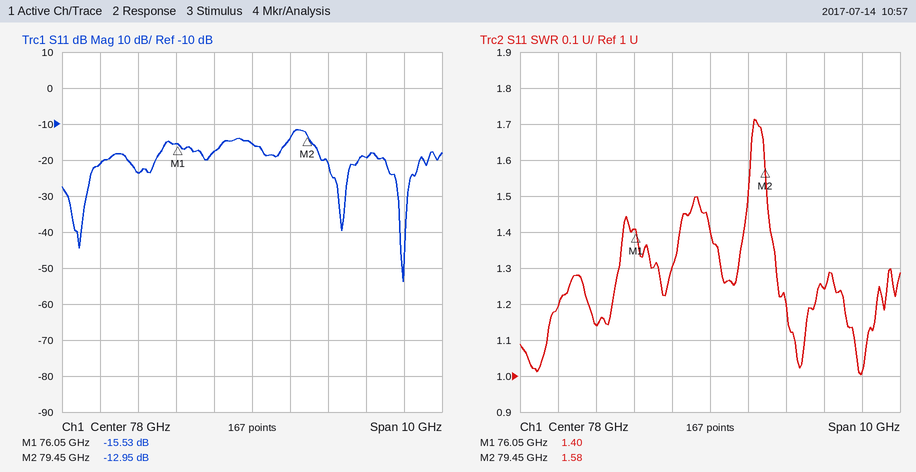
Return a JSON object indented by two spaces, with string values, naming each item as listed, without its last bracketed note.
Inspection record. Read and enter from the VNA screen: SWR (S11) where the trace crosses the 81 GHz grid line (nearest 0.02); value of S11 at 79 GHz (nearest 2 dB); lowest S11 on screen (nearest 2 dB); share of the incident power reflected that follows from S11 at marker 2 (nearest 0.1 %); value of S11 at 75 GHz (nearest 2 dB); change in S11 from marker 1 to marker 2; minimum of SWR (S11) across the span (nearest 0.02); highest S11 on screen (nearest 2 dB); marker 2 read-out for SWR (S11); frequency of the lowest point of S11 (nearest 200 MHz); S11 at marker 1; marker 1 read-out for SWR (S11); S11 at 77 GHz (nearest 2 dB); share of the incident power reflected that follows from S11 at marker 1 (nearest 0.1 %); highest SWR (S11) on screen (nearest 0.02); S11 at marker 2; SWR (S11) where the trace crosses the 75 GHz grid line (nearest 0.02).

{
  "SWR (S11) where the trace crosses the 81 GHz grid line": "1.24",
  "value of S11 at 79 GHz": "-14 dB",
  "lowest S11 on screen": "-54 dB",
  "share of the incident power reflected that follows from S11 at marker 2": "5.1 %",
  "value of S11 at 75 GHz": "-24 dB",
  "change in S11 from marker 1 to marker 2": "2.58 dB",
  "minimum of SWR (S11) across the span": "1.00",
  "highest S11 on screen": "-12 dB",
  "marker 2 read-out for SWR": "1.58",
  "frequency of the lowest point of S11": "82.0 GHz",
  "S11 at marker 1": "-15.53 dB",
  "marker 1 read-out for SWR": "1.40",
  "S11 at 77 GHz": "-18 dB",
  "share of the incident power reflected that follows from S11 at marker 1": "2.8 %",
  "highest SWR (S11) on screen": "1.72",
  "S11 at marker 2": "-12.95 dB",
  "SWR (S11) where the trace crosses the 75 GHz grid line": "1.14"
}
